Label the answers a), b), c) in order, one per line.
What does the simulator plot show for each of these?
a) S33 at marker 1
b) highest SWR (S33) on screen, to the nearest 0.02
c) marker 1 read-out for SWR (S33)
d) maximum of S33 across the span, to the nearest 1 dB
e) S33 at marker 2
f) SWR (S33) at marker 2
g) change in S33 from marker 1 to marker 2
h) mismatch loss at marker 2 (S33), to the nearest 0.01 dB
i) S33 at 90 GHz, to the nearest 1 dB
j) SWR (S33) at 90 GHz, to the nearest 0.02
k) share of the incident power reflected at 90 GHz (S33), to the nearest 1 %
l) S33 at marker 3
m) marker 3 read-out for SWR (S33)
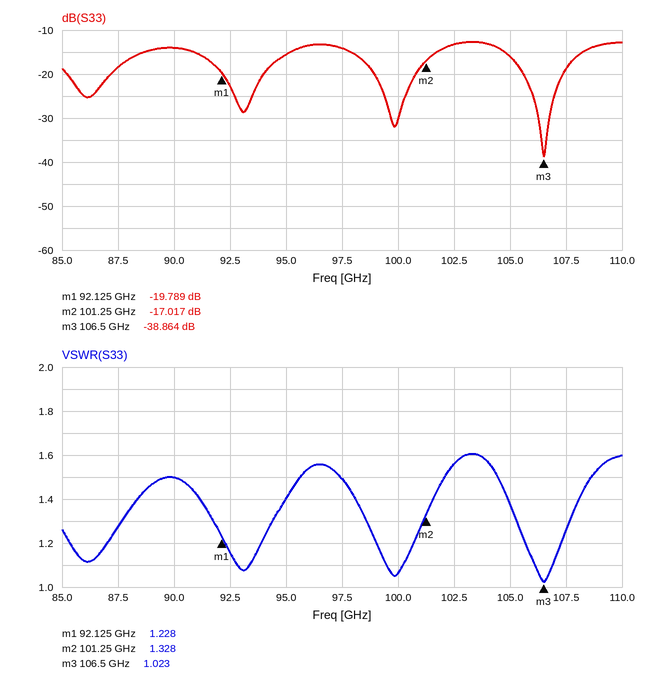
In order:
a) -19.789 dB
b) 1.60
c) 1.228
d) -13 dB
e) -17.017 dB
f) 1.328
g) 2.772 dB
h) 0.09 dB
i) -14 dB
j) 1.50
k) 4 %
l) -38.864 dB
m) 1.023
